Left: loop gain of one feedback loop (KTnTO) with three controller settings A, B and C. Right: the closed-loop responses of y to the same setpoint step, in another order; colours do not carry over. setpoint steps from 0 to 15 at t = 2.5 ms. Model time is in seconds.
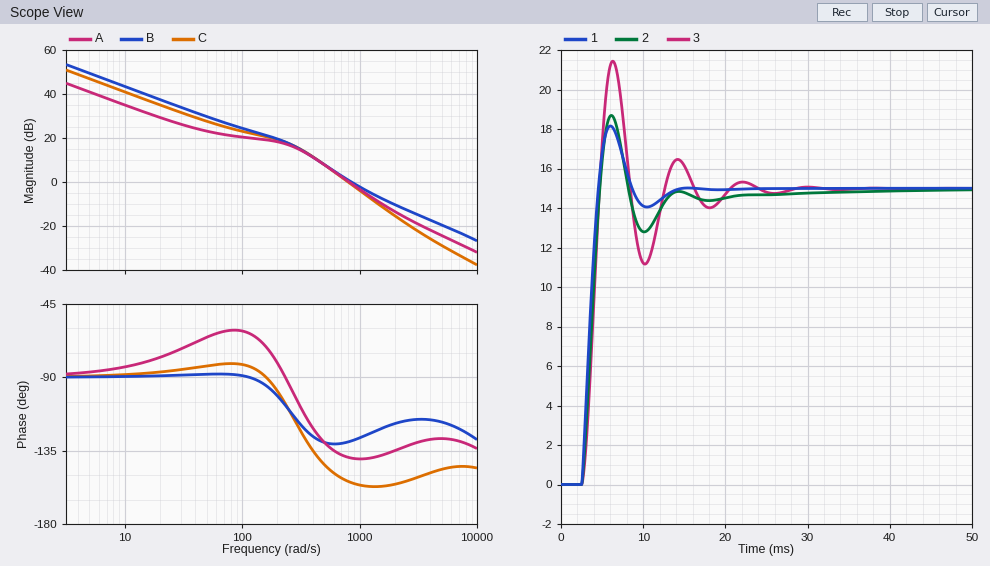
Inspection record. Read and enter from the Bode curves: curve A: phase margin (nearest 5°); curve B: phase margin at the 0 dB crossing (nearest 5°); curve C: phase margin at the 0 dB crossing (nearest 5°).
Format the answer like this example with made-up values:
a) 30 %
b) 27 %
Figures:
a) 40°
b) 50°
c) 25°
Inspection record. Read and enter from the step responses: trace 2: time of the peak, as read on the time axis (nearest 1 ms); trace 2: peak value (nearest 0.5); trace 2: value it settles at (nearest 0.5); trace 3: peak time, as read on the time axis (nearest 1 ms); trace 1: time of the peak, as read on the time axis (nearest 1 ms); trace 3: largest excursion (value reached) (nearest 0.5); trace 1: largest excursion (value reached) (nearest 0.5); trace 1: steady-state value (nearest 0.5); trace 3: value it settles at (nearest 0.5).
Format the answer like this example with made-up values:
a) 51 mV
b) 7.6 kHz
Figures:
a) 6 ms
b) 18.5
c) 15.0
d) 6 ms
e) 6 ms
f) 21.5
g) 18.0
h) 15.0
i) 15.0
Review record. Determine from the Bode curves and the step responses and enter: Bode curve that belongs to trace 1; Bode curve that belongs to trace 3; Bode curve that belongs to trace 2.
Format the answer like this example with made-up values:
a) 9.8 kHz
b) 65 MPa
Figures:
a) B
b) C
c) A
